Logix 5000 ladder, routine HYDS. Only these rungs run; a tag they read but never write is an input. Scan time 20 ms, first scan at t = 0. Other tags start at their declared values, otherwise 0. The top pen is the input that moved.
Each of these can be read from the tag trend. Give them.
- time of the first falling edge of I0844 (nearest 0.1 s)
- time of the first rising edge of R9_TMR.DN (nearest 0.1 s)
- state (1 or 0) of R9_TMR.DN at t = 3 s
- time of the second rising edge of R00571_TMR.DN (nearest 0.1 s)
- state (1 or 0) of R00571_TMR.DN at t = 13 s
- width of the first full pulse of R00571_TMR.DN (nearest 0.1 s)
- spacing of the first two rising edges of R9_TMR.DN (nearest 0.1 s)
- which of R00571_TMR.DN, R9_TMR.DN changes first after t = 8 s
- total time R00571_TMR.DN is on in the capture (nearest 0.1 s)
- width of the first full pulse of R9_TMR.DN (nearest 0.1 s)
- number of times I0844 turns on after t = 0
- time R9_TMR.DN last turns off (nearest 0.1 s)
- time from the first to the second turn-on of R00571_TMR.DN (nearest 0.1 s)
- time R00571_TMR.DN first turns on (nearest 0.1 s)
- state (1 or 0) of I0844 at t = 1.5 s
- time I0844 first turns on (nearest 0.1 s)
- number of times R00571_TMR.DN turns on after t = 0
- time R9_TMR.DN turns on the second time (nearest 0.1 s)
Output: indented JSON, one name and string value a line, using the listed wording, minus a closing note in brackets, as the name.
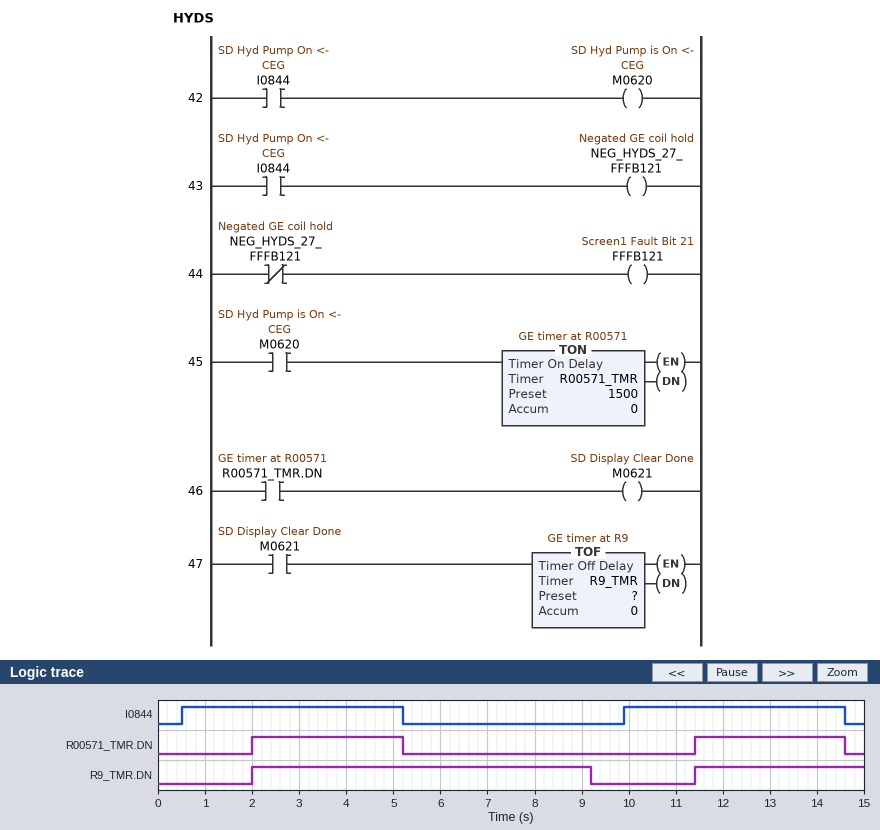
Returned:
{
  "time of the first falling edge of I0844": "5.2 s",
  "time of the first rising edge of R9_TMR.DN": "2.0 s",
  "state (1 or 0) of R9_TMR.DN at t = 3 s": "1",
  "time of the second rising edge of R00571_TMR.DN": "11.4 s",
  "state (1 or 0) of R00571_TMR.DN at t = 13 s": "1",
  "width of the first full pulse of R00571_TMR.DN": "3.2 s",
  "spacing of the first two rising edges of R9_TMR.DN": "9.4 s",
  "which of R00571_TMR.DN, R9_TMR.DN changes first after t = 8 s": "R9_TMR.DN",
  "total time R00571_TMR.DN is on in the capture": "6.4 s",
  "width of the first full pulse of R9_TMR.DN": "7.2 s",
  "number of times I0844 turns on after t = 0": "2",
  "time R9_TMR.DN last turns off": "9.2 s",
  "time from the first to the second turn-on of R00571_TMR.DN": "9.4 s",
  "time R00571_TMR.DN first turns on": "2.0 s",
  "state (1 or 0) of I0844 at t = 1.5 s": "1",
  "time I0844 first turns on": "0.5 s",
  "number of times R00571_TMR.DN turns on after t = 0": "2",
  "time R9_TMR.DN turns on the second time": "11.4 s"
}
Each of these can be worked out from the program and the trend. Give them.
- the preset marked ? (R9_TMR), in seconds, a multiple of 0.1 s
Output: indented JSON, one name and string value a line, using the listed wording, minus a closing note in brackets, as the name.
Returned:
{
  "the preset marked ? (R9_TMR), in seconds, a multiple of 0.1 s": "4.0 s"
}
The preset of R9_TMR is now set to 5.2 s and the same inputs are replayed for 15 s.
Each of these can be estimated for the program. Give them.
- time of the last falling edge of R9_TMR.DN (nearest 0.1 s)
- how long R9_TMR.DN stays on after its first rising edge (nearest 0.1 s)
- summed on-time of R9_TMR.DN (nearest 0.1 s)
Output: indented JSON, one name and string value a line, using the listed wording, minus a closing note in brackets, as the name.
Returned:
{
  "time of the last falling edge of R9_TMR.DN": "10.4 s",
  "how long R9_TMR.DN stays on after its first rising edge": "8.4 s",
  "summed on-time of R9_TMR.DN": "12.0 s"
}
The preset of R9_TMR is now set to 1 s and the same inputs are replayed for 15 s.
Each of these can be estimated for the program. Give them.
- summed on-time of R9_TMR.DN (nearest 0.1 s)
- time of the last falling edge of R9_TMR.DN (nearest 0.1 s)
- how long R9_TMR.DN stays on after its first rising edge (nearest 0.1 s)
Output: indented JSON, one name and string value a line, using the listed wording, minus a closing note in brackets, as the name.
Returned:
{
  "summed on-time of R9_TMR.DN": "7.8 s",
  "time of the last falling edge of R9_TMR.DN": "6.2 s",
  "how long R9_TMR.DN stays on after its first rising edge": "4.2 s"
}
